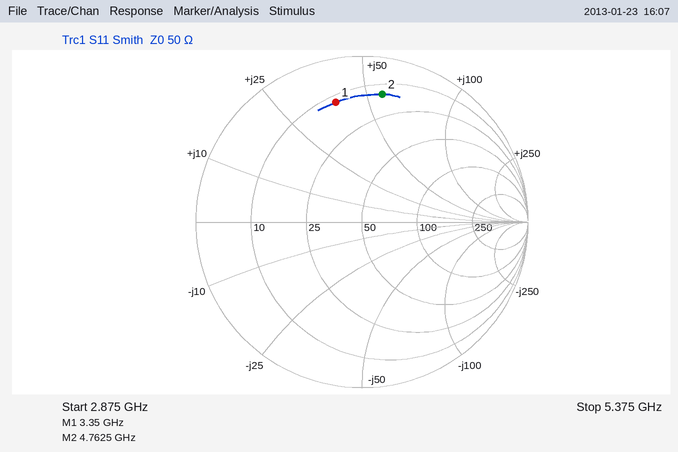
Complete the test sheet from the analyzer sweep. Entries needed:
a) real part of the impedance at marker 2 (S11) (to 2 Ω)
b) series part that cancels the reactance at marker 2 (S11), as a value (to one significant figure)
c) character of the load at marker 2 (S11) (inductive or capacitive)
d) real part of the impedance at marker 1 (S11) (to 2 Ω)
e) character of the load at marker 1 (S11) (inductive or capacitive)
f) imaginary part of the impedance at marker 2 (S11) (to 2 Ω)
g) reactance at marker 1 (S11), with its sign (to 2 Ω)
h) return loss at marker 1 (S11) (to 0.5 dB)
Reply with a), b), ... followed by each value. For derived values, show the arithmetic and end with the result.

a) 14 Ω
b) C = 1/(2π × 4.7625 GHz × 56 Ω) ≈ 597 fF, so 600 fF to one significant figure
c) inductive
d) 12 Ω
e) inductive
f) +56 Ω
g) +38 Ω
h) 2.5 dB
